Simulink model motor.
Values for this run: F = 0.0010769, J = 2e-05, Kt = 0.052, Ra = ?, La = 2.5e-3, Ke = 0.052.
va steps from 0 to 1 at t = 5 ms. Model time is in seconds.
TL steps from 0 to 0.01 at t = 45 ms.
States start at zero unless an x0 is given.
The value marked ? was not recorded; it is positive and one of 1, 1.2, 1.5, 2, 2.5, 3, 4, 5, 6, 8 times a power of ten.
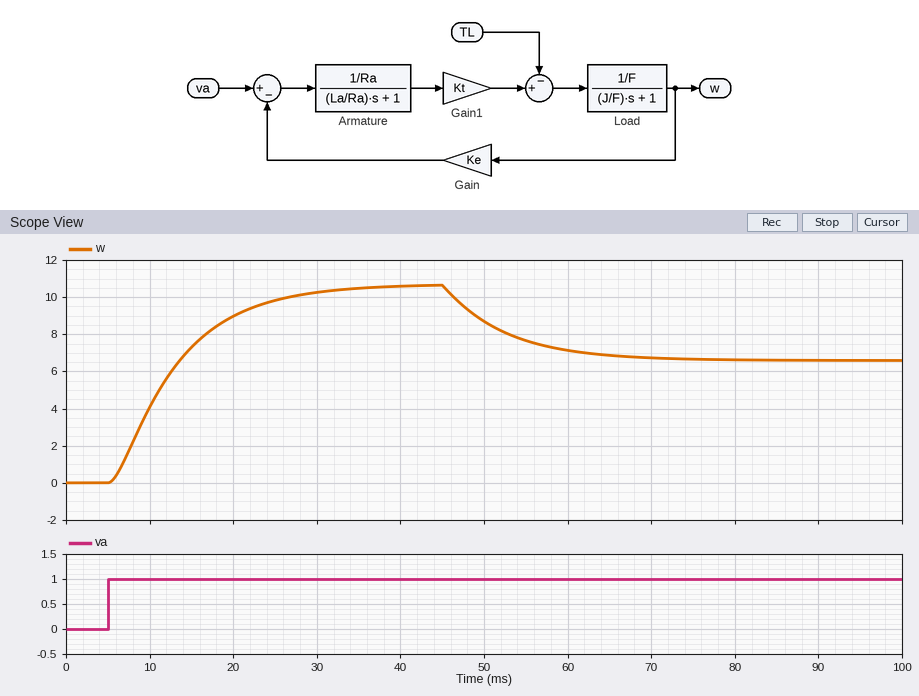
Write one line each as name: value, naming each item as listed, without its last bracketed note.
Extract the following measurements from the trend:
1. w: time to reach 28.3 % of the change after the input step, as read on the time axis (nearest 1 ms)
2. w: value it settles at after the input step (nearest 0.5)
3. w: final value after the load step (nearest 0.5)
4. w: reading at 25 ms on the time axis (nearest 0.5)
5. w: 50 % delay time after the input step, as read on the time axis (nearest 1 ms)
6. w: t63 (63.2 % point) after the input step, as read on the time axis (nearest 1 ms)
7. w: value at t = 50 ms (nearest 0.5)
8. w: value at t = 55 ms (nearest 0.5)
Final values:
w: time to reach 28.3 % of the change after the input step, as read on the time axis: 9 ms
w: value it settles at after the input step: 10.5
w: final value after the load step: 6.5
w: reading at 25 ms on the time axis: 10.0
w: 50 % delay time after the input step, as read on the time axis: 12 ms
w: t63 (63.2 % point) after the input step, as read on the time axis: 14 ms
w: value at t = 50 ms: 8.5
w: value at t = 55 ms: 7.5
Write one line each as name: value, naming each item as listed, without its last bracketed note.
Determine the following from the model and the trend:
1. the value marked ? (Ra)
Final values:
the value marked ?: 2
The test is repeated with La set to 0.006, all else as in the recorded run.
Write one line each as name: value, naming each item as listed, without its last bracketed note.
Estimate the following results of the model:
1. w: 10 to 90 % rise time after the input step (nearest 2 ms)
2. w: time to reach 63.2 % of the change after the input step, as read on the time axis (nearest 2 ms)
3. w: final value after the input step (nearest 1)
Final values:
w: 10 to 90 % rise time after the input step: 16 ms
w: time to reach 63.2 % of the change after the input step, as read on the time axis: 16 ms
w: final value after the input step: 11
